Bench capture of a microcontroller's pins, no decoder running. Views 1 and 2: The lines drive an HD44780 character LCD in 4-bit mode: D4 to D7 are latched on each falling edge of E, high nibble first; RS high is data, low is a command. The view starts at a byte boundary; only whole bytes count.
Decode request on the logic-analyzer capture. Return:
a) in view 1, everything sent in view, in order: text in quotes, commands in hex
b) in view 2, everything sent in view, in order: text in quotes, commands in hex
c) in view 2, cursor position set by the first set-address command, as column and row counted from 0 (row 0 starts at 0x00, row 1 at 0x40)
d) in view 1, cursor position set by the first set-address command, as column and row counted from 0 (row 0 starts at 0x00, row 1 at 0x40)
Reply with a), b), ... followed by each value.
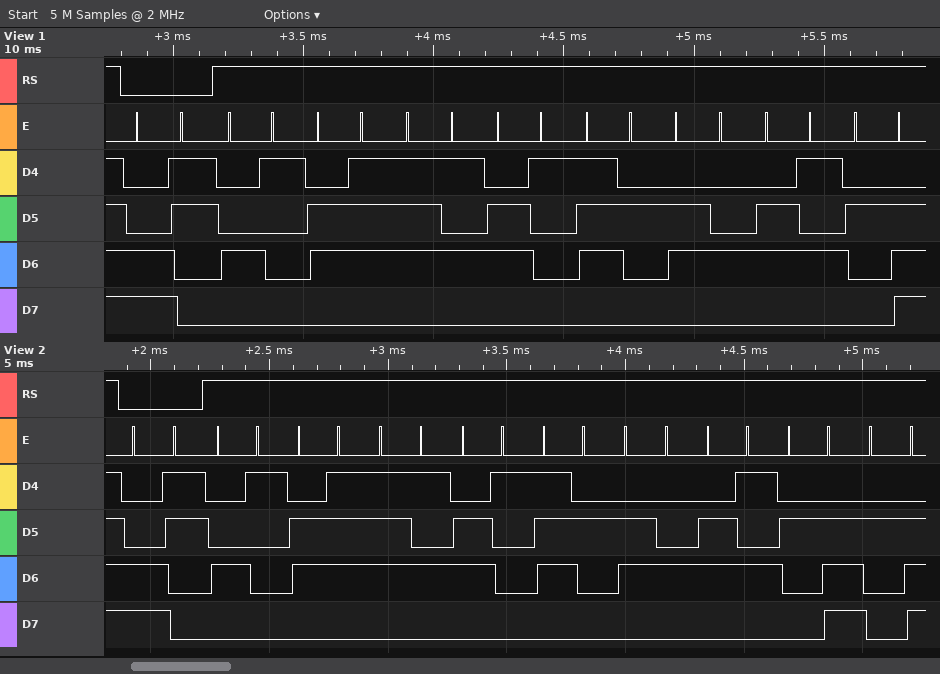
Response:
a) 0xC3 "Aguarde."
b) 0xC3 "Aguarde.."
c) column 3, row 1
d) column 3, row 1
